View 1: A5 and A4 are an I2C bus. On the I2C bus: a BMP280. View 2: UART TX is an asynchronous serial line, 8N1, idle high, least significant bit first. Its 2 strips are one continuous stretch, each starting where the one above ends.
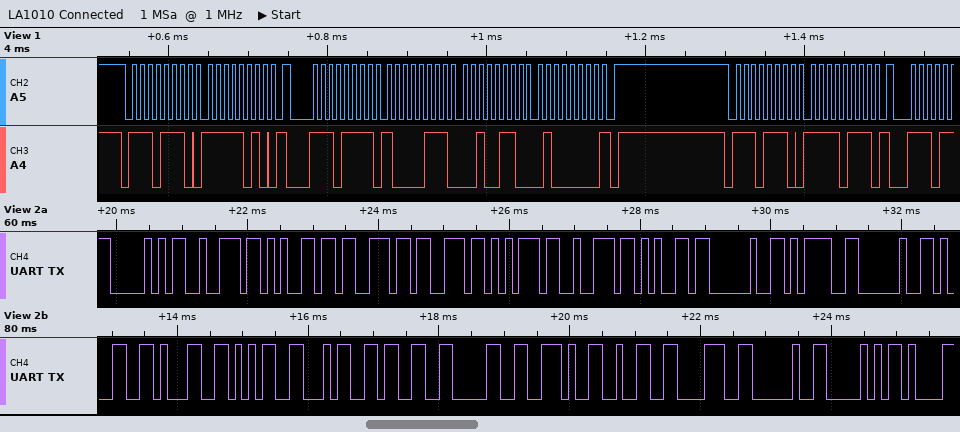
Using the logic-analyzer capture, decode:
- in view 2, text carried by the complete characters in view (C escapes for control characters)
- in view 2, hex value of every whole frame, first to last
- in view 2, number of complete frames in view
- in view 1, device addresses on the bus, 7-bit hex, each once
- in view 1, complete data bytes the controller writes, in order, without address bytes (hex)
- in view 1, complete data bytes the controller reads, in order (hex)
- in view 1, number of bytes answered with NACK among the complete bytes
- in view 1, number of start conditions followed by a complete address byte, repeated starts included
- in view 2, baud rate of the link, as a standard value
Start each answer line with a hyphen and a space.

- "Pressure = 115430.28 P"
- 0x50 0x72 0x65 0x73 0x73 0x75 0x72 0x65 0x20 0x3D 0x20 0x31 0x31 0x35 0x34 0x33 0x30 0x2E 0x32 0x38 0x20 0x50
- 22
- 0x77
- FA F7
- 87 26 40
- 1
- 3
- 9600 baud
